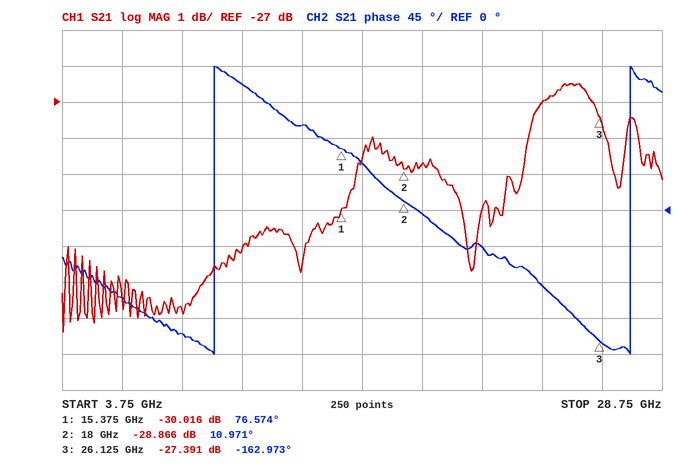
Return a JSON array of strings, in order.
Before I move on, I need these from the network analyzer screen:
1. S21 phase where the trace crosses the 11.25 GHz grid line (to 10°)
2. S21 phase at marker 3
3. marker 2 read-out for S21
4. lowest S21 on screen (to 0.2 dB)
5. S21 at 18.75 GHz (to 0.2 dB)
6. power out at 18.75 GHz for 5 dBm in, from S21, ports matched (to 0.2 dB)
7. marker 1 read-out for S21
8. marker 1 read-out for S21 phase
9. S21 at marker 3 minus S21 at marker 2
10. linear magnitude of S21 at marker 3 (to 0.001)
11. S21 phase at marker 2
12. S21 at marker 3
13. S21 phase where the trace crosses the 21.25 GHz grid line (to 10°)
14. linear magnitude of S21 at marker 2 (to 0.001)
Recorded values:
["160°", "-162.973°", "-28.866 dB", "-33.4 dB", "-28.8 dB", "-23.8 dBm", "-30.016 dB", "76.574°", "1.475 dB", "0.043", "10.971°", "-27.391 dB", "-50°", "0.036"]
